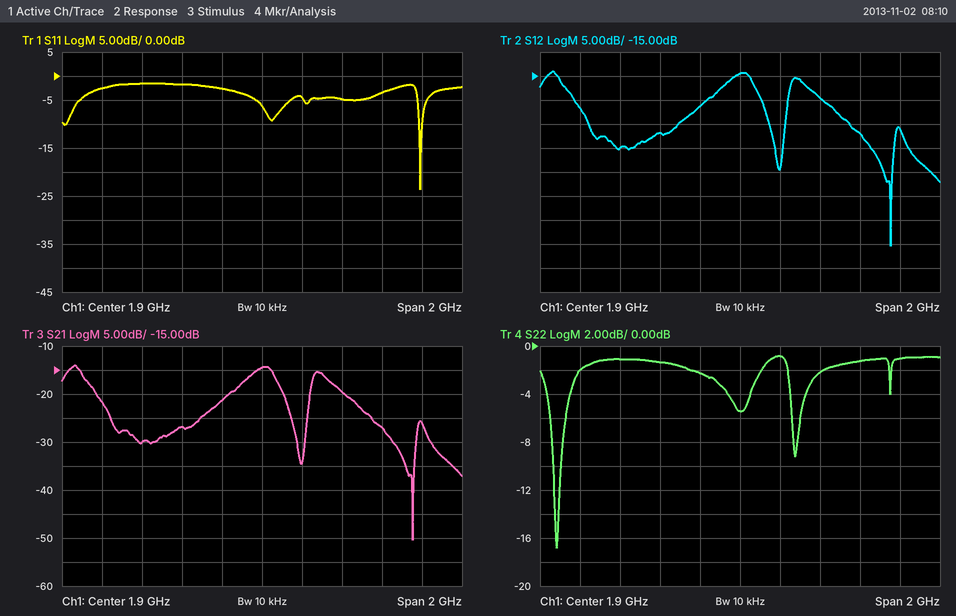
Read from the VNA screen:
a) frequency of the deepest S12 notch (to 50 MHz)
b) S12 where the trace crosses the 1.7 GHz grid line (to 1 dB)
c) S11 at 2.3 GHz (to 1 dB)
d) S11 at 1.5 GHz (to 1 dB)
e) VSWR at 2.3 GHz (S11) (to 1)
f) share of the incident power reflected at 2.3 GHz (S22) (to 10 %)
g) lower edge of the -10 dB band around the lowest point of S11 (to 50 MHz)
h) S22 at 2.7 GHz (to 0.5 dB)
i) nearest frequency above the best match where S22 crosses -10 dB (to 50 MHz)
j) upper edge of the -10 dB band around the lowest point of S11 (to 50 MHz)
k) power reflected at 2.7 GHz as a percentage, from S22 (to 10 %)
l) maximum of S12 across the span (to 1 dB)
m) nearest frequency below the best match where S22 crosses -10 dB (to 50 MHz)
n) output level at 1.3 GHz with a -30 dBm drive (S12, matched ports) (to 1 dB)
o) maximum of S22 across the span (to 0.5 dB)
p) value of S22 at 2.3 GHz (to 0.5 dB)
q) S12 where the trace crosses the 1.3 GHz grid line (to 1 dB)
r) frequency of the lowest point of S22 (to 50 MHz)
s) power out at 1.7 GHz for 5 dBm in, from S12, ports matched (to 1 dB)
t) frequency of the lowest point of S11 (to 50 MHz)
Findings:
2.65 GHz
-21 dB
-5 dB
-2 dB
4
60 %
2.70 GHz
-1.0 dB
1.00 GHz
2.70 GHz
80 %
-14 dB
950 MHz
-60 dBm
-1.0 dB
-2.0 dB
-30 dB
1.00 GHz
-16 dBm
2.70 GHz
